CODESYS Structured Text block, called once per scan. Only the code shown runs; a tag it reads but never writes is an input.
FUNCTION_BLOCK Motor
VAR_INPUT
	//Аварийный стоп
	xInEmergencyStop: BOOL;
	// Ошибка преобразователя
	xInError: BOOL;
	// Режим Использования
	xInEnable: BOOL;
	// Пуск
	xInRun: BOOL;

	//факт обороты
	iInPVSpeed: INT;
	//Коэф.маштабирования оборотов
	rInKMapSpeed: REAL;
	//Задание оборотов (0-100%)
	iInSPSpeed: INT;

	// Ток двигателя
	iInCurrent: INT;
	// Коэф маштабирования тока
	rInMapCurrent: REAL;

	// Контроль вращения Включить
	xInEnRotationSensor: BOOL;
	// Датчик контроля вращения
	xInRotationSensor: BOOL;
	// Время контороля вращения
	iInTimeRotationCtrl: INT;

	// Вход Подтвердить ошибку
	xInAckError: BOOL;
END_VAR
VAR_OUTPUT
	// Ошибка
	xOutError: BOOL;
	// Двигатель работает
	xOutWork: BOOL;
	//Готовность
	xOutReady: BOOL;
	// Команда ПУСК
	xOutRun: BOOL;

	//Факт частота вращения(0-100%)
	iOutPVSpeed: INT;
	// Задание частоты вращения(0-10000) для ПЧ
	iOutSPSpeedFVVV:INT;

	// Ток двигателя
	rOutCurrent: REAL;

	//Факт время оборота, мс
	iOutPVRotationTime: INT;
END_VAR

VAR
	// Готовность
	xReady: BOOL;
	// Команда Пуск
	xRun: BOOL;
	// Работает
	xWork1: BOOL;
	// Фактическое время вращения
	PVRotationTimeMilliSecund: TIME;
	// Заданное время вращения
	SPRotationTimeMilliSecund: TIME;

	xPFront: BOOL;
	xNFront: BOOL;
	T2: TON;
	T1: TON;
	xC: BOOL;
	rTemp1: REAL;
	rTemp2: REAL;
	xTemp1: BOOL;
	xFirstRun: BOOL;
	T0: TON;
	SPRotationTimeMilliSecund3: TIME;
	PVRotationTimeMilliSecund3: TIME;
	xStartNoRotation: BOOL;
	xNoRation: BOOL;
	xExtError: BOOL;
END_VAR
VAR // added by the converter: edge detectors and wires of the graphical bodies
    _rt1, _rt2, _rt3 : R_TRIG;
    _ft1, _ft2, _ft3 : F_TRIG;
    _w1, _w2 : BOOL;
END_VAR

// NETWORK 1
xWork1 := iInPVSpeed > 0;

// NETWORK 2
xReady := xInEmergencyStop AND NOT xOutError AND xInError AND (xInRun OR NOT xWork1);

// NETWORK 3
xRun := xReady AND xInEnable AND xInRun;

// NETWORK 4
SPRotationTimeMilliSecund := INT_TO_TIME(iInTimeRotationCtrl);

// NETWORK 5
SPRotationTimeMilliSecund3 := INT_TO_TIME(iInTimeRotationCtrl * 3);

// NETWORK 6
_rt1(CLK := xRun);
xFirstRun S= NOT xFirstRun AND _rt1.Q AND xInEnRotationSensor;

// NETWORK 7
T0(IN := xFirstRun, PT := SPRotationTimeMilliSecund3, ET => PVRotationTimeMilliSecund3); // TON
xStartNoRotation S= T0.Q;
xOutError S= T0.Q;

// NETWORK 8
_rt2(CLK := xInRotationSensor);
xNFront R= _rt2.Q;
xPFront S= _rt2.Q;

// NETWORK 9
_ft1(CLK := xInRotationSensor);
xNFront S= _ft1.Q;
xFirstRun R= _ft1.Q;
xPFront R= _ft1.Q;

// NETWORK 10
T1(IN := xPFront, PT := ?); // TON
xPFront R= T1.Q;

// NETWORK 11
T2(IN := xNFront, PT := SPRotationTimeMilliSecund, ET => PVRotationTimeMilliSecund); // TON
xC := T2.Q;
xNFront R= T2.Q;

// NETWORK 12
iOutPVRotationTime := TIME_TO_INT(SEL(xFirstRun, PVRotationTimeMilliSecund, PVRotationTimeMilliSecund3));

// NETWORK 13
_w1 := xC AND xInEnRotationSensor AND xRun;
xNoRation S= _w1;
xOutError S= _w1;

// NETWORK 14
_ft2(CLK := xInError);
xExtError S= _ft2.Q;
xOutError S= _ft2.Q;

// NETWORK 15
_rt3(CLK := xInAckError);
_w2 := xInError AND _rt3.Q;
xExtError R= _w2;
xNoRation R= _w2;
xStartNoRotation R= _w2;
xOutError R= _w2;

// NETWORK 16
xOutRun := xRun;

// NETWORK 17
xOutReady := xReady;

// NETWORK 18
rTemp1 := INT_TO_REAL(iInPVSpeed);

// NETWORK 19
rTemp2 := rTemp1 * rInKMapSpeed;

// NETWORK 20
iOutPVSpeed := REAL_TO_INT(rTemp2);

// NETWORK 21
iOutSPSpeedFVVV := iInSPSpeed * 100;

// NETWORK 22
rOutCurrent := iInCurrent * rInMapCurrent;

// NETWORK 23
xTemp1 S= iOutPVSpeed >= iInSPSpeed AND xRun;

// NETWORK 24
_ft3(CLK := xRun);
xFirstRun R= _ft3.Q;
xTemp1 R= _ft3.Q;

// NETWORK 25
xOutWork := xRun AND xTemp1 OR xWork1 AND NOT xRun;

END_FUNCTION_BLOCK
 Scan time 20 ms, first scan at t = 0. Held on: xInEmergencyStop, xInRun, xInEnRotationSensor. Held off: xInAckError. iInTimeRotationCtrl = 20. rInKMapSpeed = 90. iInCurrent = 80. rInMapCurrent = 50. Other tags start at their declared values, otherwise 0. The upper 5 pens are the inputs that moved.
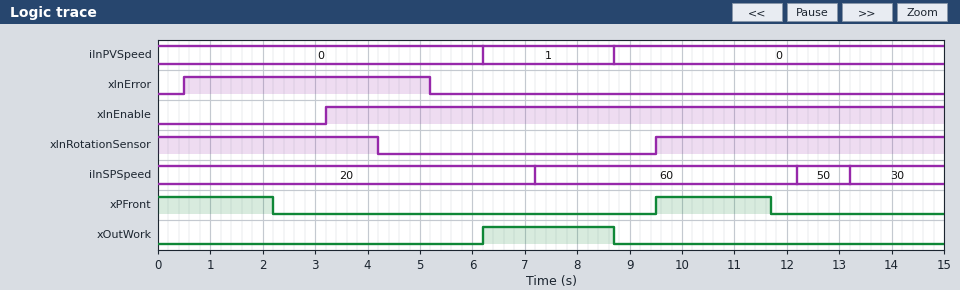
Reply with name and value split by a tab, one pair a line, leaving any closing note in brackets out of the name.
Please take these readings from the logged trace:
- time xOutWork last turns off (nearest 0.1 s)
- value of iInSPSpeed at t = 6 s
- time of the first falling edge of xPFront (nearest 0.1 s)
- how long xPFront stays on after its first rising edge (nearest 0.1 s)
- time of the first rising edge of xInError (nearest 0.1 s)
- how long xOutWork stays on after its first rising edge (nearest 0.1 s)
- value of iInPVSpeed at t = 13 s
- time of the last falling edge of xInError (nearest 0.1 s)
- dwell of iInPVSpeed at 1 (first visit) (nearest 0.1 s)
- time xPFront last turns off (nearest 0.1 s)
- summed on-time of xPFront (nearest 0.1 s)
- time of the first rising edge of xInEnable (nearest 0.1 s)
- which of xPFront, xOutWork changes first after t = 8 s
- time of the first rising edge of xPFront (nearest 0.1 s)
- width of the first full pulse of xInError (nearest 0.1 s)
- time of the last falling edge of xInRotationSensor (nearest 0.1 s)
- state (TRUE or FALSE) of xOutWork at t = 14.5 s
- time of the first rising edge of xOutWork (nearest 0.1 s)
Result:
time xOutWork last turns off	8.7 s
value of iInSPSpeed at t = 6 s	20
time of the first falling edge of xPFront	2.2 s
how long xPFront stays on after its first rising edge	2.2 s
time of the first rising edge of xInError	0.5 s
how long xOutWork stays on after its first rising edge	2.5 s
value of iInPVSpeed at t = 13 s	0
time of the last falling edge of xInError	5.2 s
dwell of iInPVSpeed at 1 (first visit)	2.5 s
time xPFront last turns off	11.7 s
summed on-time of xPFront	4.4 s
time of the first rising edge of xInEnable	3.2 s
which of xPFront, xOutWork changes first after t = 8 s	xOutWork
time of the first rising edge of xPFront	9.5 s
width of the first full pulse of xInError	4.7 s
time of the last falling edge of xInRotationSensor	4.2 s
state (TRUE or FALSE) of xOutWork at t = 14.5 s	FALSE
time of the first rising edge of xOutWork	6.2 s
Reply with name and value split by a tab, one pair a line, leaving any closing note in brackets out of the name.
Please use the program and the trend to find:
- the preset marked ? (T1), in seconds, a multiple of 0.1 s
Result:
the preset marked ? (T1), in seconds, a multiple of 0.1 s	2.2 s
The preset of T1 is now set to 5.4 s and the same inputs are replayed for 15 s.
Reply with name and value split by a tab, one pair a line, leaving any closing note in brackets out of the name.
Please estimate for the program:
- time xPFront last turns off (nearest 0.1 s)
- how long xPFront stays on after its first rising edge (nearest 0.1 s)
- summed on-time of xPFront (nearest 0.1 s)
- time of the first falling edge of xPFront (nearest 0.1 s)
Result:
time xPFront last turns off	14.9 s
how long xPFront stays on after its first rising edge	5.4 s
summed on-time of xPFront	9.6 s
time of the first falling edge of xPFront	4.2 s
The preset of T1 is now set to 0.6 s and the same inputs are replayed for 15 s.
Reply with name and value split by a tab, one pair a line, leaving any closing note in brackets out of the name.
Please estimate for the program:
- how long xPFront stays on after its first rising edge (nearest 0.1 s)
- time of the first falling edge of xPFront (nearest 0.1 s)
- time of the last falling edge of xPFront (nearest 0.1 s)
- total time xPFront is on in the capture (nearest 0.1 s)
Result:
how long xPFront stays on after its first rising edge	0.6 s
time of the first falling edge of xPFront	0.6 s
time of the last falling edge of xPFront	10.1 s
total time xPFront is on in the capture	1.2 s
